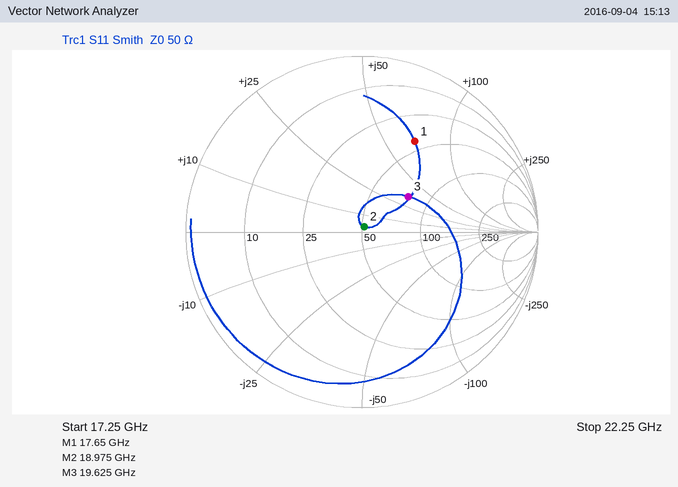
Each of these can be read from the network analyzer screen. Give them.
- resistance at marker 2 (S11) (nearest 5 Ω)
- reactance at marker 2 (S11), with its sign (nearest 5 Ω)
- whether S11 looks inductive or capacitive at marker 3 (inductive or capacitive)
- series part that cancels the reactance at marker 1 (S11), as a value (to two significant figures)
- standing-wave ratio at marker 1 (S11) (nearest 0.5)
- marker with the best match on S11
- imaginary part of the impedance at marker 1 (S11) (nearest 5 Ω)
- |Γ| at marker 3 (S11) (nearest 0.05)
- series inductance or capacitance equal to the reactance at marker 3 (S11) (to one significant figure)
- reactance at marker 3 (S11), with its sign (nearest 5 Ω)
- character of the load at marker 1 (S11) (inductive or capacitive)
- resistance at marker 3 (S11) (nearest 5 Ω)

50 Ω
+5 Ω
inductive
130 fF
4.0
marker 2
+70 Ω
0.35
300 pH
+35 Ω
inductive
75 Ω
